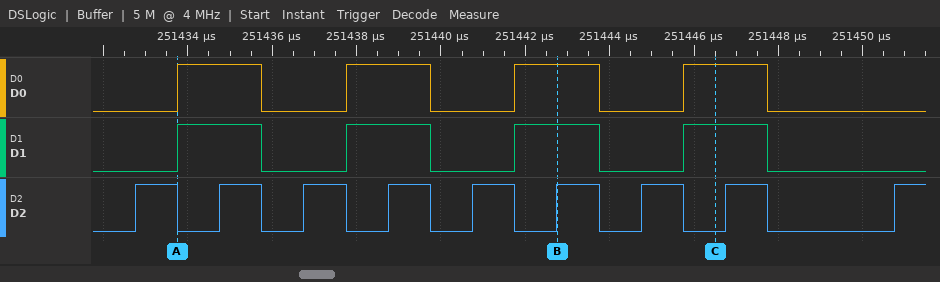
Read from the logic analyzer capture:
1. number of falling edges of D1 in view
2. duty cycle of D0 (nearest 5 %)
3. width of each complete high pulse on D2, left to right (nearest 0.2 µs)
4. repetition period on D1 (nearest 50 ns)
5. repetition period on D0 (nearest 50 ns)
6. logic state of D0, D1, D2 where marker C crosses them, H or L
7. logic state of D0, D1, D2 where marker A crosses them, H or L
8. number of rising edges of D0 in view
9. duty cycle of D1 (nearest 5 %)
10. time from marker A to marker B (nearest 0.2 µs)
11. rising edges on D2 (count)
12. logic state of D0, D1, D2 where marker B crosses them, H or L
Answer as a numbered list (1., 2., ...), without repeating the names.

1. 4
2. 50 %
3. 1 µs, 1 µs, 1 µs, 1 µs, 1 µs, 1 µs, 1 µs, 1 µs
4. 4000 ns
5. 4000 ns
6. D0=H, D1=H, D2=L
7. D0=H, D1=H, D2=L
8. 4
9. 50 %
10. 9 µs
11. 9
12. D0=H, D1=H, D2=H
